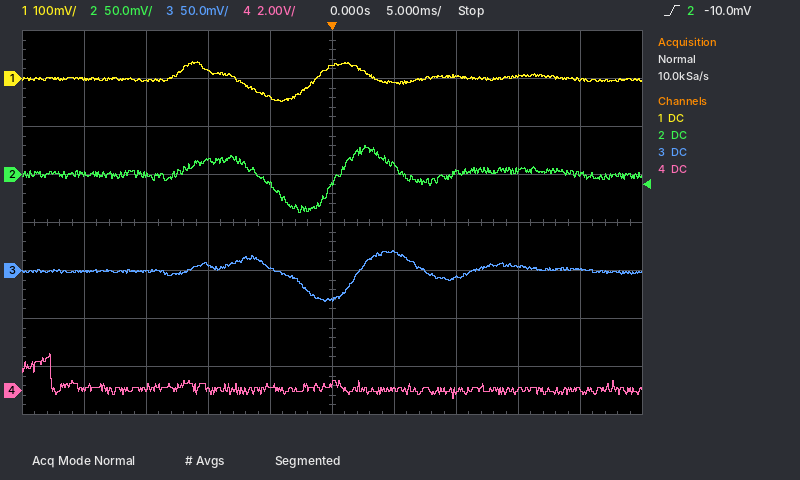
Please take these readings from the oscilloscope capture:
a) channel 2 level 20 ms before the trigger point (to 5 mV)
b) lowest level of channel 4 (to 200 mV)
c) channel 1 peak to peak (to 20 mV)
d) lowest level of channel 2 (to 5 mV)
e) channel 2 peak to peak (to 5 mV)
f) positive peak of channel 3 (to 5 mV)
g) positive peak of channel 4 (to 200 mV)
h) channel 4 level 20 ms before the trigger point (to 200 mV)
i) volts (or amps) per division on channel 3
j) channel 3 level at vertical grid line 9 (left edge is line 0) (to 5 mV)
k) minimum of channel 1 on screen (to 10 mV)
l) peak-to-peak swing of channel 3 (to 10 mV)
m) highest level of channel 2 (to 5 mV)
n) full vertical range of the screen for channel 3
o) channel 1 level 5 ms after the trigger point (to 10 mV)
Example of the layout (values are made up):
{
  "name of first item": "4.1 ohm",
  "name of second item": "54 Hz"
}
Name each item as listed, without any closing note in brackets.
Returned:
{
  "channel 2 level 20 ms before the trigger point": "0 mV",
  "lowest level of channel 4": "-400 mV",
  "channel 1 peak to peak": "80 mV",
  "lowest level of channel 2": "-40 mV",
  "channel 2 peak to peak": "70 mV",
  "positive peak of channel 3": "20 mV",
  "positive peak of channel 4": "1.6 V",
  "channel 4 level 20 ms before the trigger point": "0.0 V",
  "volts (or amps) per division on channel 3": "50 mV",
  "channel 3 level at vertical grid line 9 (left edge is line 0)": "0 mV",
  "minimum of channel 1 on screen": "-50 mV",
  "peak-to-peak swing of channel 3": "50 mV",
  "highest level of channel 2": "30 mV",
  "full vertical range of the screen for channel 3": "400 mV",
  "channel 1 level 5 ms after the trigger point": "-10 mV"
}
